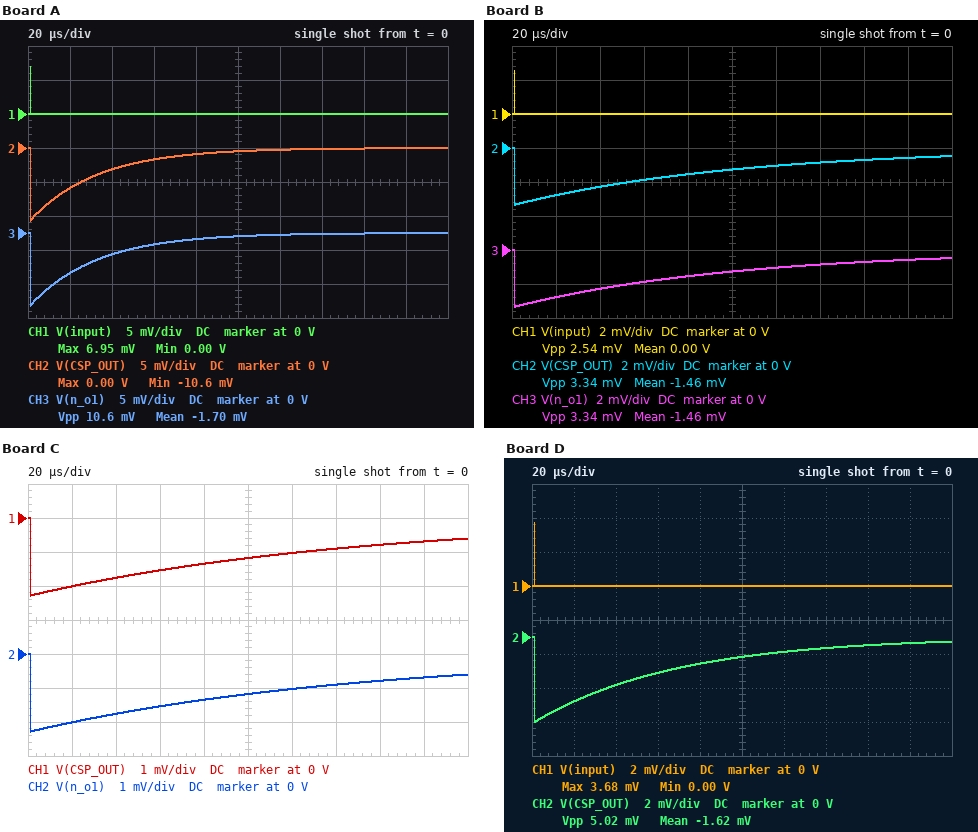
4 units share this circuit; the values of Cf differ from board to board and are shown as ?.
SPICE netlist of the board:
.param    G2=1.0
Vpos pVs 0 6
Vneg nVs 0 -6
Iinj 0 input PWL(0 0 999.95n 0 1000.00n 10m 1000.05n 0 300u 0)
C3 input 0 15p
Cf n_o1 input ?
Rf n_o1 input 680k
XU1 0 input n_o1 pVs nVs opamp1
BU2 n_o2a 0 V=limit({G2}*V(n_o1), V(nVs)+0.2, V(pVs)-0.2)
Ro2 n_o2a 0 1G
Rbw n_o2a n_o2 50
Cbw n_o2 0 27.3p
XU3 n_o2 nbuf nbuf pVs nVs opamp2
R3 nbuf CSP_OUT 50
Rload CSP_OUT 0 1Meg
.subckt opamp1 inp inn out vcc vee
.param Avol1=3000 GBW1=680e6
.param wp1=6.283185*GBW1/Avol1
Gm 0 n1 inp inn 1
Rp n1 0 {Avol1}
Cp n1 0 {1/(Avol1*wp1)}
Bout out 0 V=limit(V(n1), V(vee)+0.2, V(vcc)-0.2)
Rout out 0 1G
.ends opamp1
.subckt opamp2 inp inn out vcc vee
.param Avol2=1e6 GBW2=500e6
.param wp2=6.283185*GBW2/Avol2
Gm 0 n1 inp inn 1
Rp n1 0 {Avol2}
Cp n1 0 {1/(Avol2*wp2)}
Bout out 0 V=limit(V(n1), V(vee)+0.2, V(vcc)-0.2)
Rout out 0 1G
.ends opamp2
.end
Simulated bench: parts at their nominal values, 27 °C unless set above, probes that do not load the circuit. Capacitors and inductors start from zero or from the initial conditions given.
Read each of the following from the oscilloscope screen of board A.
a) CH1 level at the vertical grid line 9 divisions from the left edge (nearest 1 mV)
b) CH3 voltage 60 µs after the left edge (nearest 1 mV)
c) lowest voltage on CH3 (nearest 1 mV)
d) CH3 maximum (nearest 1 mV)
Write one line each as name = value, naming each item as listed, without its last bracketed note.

CH1 level at the vertical grid line 9 divisions from the left edge = 0 V
CH3 voltage 60 µs after the left edge = -2 mV
lowest voltage on CH3 = -11 mV
CH3 maximum = 0 V
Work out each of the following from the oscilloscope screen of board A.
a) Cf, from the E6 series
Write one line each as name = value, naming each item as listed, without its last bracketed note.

Cf, from the E6 series = 47 pF
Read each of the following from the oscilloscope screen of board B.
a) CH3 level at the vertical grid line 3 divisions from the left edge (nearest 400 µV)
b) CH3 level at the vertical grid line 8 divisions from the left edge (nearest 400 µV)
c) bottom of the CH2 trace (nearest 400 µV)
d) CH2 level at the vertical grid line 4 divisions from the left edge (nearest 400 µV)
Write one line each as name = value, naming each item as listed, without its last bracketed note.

CH3 level at the vertical grid line 3 divisions from the left edge = -2.0 mV
CH3 level at the vertical grid line 8 divisions from the left edge = -800 µV
bottom of the CH2 trace = -3.2 mV
CH2 level at the vertical grid line 4 divisions from the left edge = -1.6 mV
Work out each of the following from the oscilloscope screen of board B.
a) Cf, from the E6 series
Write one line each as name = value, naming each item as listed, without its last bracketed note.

Cf, from the E6 series = 150 pF
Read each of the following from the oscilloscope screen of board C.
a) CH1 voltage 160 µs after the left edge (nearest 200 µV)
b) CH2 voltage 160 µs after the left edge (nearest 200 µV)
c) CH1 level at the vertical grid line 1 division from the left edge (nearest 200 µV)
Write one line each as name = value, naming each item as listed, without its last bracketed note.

CH1 voltage 160 µs after the left edge = -800 µV
CH2 voltage 160 µs after the left edge = -800 µV
CH1 level at the vertical grid line 1 division from the left edge = -2.0 mV
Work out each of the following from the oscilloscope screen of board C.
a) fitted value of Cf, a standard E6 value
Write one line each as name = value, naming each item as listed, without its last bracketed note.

fitted value of Cf, a standard E6 value = 220 pF
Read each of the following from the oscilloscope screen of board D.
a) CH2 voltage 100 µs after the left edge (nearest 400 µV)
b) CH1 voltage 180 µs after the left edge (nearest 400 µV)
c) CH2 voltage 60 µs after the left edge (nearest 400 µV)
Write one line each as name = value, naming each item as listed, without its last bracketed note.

CH2 voltage 100 µs after the left edge = -1.2 mV
CH1 voltage 180 µs after the left edge = 0 V
CH2 voltage 60 µs after the left edge = -2.0 mV
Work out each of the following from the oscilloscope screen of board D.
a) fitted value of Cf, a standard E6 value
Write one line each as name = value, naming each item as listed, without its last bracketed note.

fitted value of Cf, a standard E6 value = 100 pF
